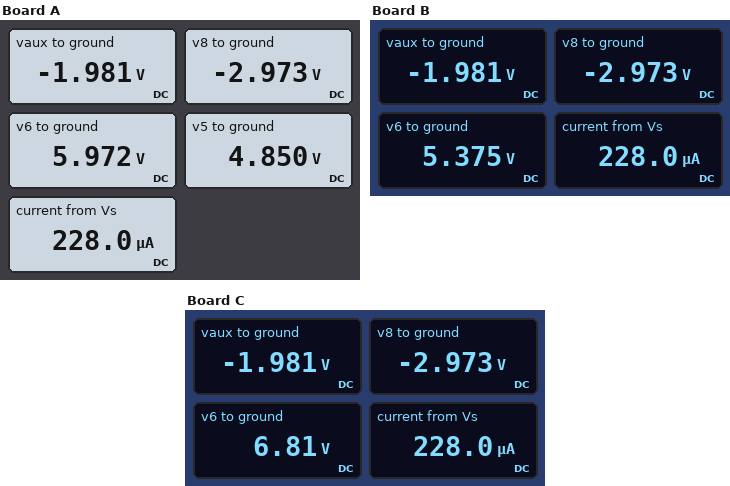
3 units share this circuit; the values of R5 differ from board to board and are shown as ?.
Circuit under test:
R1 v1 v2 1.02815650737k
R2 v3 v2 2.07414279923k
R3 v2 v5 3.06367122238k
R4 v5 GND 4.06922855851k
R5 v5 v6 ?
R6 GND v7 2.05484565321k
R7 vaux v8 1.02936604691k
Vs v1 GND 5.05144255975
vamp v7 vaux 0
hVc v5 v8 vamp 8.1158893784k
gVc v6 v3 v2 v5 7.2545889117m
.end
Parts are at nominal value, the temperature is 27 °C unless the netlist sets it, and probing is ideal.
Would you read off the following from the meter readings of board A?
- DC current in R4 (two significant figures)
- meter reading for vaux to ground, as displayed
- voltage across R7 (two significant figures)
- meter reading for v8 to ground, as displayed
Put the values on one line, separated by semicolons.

1.2 mA; -1.981 V; 990 mV; -2.973 V
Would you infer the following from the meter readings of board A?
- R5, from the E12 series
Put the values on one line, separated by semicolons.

4.7 kΩ
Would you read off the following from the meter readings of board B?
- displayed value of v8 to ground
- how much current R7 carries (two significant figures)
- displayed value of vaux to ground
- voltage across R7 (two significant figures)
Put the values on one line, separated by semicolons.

-2.973 V; 960 µA; -1.981 V; 990 mV
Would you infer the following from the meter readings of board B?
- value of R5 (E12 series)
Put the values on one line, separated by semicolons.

2.2 kΩ
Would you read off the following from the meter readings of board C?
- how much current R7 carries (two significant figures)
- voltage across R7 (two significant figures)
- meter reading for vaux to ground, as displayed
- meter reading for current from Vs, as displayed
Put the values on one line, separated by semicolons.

960 µA; 990 mV; -1.981 V; 228.0 µA
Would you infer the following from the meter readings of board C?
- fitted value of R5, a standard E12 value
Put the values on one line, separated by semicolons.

8.2 kΩ
